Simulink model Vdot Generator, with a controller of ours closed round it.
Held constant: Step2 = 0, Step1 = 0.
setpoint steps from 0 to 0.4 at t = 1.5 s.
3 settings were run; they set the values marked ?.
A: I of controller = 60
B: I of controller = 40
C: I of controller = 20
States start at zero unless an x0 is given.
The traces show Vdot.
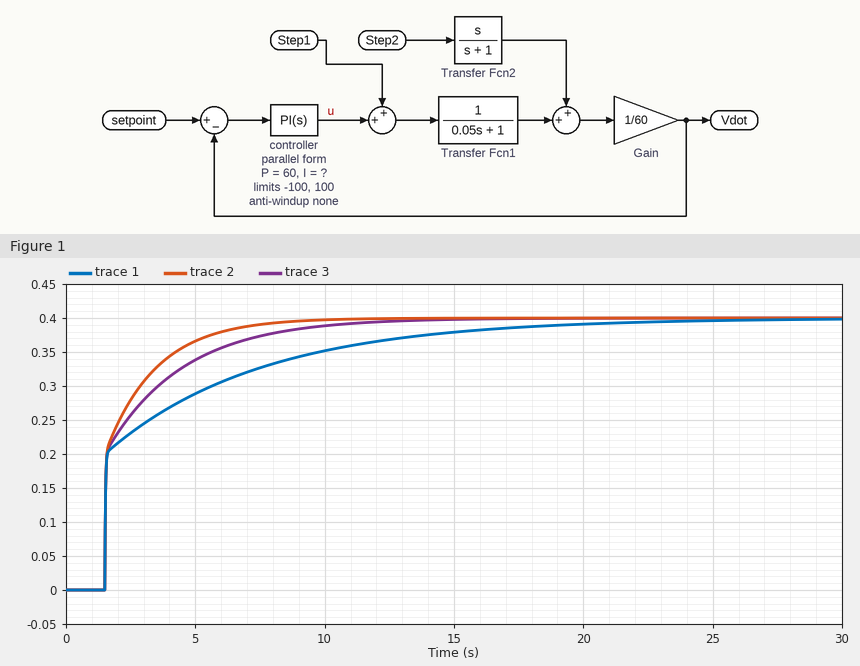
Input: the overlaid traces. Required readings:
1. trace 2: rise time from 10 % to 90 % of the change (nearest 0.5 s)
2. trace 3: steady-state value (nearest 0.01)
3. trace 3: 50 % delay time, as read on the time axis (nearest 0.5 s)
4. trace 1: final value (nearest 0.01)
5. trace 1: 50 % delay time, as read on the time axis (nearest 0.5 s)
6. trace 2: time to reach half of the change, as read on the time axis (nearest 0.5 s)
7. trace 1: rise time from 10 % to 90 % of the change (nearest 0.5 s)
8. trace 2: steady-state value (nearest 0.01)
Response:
3.0 s
0.40
1.5 s
0.40
1.5 s
1.5 s
9.5 s
0.40
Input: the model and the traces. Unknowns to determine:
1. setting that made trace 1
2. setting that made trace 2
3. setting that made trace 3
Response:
C
A
B
